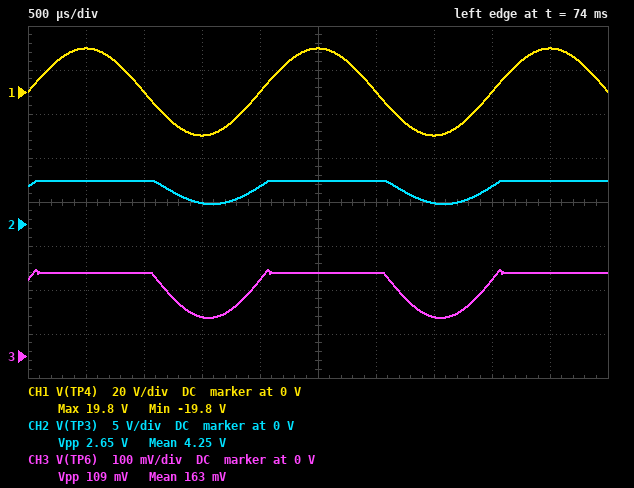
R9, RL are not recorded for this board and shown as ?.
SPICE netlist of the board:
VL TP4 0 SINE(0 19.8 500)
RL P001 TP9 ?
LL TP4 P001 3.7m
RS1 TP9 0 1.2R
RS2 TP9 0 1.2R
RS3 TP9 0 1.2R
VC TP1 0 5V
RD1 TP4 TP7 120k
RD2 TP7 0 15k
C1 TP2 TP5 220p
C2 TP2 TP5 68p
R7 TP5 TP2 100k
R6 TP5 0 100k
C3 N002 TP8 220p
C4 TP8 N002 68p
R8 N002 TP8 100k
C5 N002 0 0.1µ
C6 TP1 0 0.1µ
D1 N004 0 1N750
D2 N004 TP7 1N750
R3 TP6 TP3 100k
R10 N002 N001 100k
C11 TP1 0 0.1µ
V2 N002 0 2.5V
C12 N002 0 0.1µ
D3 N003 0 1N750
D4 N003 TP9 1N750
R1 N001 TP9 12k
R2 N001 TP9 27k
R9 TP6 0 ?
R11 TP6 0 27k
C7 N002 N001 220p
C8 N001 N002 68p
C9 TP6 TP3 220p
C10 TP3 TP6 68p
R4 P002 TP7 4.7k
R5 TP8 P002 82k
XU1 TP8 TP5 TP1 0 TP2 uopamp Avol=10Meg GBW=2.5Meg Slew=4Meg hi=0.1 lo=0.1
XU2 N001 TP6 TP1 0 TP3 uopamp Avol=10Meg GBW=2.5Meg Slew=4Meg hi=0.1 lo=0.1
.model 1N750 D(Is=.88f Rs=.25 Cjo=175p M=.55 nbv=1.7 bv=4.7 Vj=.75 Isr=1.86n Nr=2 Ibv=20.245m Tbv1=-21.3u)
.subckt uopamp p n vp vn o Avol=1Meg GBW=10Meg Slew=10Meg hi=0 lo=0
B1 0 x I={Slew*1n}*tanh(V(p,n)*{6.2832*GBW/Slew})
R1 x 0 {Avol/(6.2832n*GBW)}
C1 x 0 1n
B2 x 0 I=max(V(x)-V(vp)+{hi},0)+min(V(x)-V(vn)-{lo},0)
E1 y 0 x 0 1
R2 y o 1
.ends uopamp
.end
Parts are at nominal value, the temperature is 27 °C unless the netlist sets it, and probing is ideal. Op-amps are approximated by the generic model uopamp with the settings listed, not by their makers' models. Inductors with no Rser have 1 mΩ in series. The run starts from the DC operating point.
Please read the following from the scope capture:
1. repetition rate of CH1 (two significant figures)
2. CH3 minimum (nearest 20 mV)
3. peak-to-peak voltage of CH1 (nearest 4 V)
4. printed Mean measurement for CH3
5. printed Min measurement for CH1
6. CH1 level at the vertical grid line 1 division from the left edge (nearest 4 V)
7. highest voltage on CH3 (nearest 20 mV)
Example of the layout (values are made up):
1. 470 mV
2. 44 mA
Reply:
1. 500 Hz
2. 80 mV
3. 40 V
4. 163 mV
5. -19.8 V
6. 20 V
7. 200 mV
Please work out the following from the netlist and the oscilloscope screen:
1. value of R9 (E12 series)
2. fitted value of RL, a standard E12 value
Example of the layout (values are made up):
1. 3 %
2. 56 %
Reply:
1. 4.7 kΩ
2. 68 Ω
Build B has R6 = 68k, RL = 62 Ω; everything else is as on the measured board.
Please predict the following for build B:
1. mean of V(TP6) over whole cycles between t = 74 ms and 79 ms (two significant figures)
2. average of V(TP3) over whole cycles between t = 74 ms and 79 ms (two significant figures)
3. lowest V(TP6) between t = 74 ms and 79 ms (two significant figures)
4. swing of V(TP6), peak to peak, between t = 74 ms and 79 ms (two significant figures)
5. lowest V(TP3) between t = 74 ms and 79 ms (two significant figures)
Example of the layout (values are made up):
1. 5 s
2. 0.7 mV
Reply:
1. 150 mV
2. 4.0 V
3. 77 mV
4. 120 mV
5. 2.0 V
